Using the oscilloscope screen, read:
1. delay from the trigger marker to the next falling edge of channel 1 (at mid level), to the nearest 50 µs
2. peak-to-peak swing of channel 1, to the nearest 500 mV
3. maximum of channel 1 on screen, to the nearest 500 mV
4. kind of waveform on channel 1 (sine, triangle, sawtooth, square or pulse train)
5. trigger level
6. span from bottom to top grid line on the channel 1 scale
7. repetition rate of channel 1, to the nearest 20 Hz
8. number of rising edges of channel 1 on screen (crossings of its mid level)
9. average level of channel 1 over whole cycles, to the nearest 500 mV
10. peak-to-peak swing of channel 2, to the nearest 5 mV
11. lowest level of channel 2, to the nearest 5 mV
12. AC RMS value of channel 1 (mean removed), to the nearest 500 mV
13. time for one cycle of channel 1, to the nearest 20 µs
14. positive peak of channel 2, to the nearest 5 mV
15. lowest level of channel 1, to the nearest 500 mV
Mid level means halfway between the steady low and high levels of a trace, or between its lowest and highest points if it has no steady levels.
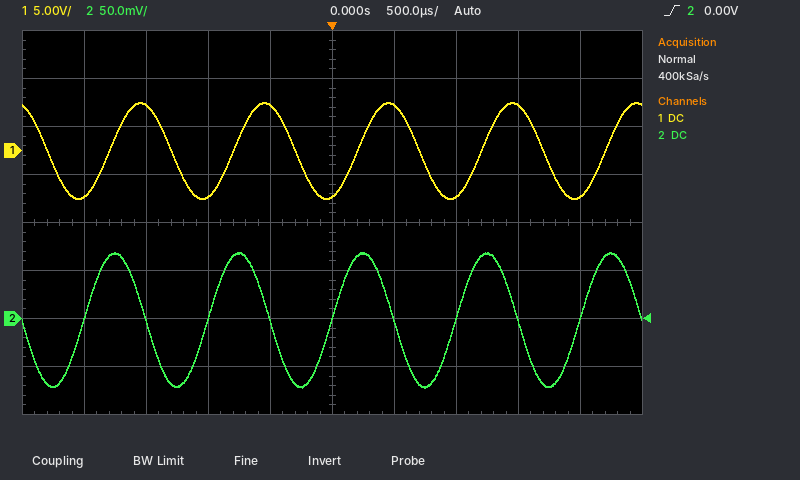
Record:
700 µs
10.0 V
5.0 V
sine
0.00 V
40 V
1.00 kHz
5
0.0 V
140 mV
-70 mV
3.5 V
1.00 ms
70 mV
-5.0 V
